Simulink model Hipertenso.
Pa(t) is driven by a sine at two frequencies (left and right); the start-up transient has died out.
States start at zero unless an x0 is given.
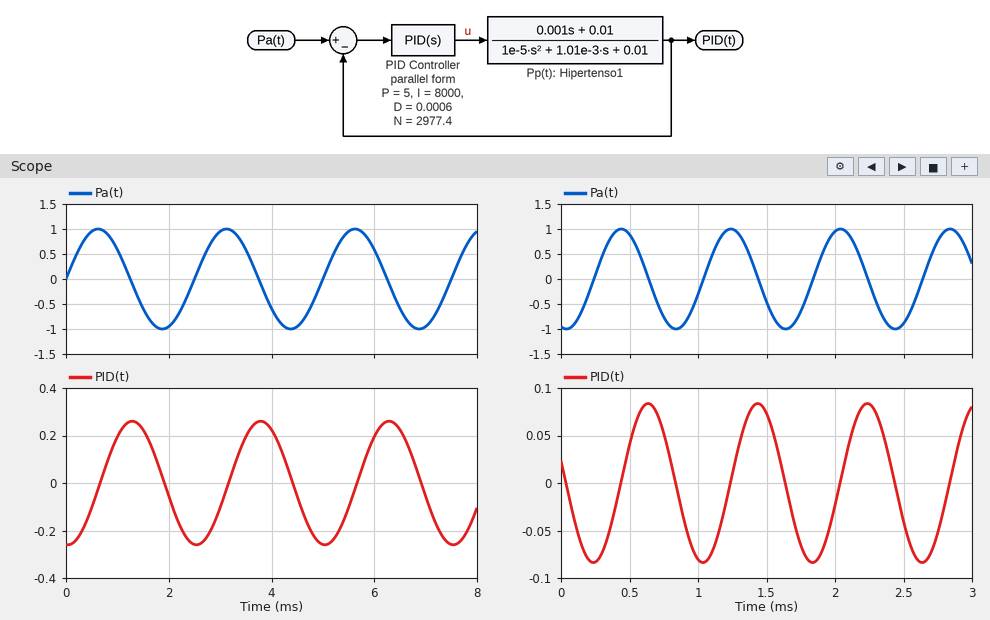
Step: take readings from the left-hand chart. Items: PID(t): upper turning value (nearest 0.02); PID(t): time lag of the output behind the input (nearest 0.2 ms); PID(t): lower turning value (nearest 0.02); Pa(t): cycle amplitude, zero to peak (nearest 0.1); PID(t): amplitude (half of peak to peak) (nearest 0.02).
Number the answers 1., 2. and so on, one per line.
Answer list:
1. 0.26
2. 0.6 ms
3. -0.26
4. 1.0
5. 0.26
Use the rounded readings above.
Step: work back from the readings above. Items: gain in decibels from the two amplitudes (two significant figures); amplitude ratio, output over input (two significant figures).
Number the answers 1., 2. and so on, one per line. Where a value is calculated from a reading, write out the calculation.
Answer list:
1. 20 log10(0.26 / 1) = -12 dB
2. 0.26 / 1 = 0.26
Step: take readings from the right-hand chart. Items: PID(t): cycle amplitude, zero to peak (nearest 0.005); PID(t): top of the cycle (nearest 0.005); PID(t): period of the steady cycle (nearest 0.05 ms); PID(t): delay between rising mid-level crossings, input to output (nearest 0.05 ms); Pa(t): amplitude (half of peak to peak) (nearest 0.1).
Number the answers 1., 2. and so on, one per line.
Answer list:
1. 0.085
2. 0.085
3. 0.80 ms
4. 0.20 ms
5. 1.0
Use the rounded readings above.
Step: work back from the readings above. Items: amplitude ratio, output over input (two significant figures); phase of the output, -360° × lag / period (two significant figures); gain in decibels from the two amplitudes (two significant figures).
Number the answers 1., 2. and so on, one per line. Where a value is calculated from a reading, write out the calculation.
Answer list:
1. 0.085 / 1 = 0.085
2. -360 × 0.2 / 0.8 = -90°
3. 20 log10(0.085 / 1) = -21 dB
